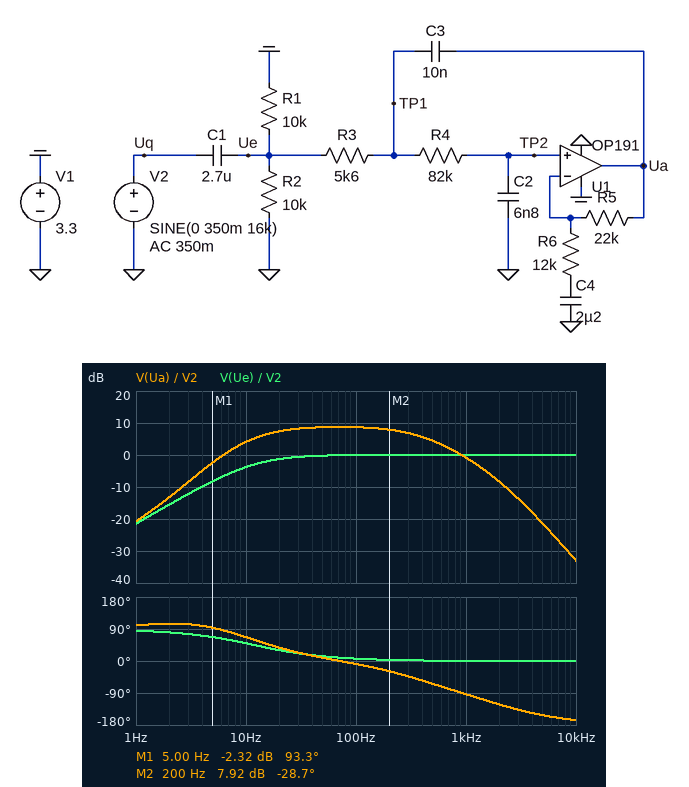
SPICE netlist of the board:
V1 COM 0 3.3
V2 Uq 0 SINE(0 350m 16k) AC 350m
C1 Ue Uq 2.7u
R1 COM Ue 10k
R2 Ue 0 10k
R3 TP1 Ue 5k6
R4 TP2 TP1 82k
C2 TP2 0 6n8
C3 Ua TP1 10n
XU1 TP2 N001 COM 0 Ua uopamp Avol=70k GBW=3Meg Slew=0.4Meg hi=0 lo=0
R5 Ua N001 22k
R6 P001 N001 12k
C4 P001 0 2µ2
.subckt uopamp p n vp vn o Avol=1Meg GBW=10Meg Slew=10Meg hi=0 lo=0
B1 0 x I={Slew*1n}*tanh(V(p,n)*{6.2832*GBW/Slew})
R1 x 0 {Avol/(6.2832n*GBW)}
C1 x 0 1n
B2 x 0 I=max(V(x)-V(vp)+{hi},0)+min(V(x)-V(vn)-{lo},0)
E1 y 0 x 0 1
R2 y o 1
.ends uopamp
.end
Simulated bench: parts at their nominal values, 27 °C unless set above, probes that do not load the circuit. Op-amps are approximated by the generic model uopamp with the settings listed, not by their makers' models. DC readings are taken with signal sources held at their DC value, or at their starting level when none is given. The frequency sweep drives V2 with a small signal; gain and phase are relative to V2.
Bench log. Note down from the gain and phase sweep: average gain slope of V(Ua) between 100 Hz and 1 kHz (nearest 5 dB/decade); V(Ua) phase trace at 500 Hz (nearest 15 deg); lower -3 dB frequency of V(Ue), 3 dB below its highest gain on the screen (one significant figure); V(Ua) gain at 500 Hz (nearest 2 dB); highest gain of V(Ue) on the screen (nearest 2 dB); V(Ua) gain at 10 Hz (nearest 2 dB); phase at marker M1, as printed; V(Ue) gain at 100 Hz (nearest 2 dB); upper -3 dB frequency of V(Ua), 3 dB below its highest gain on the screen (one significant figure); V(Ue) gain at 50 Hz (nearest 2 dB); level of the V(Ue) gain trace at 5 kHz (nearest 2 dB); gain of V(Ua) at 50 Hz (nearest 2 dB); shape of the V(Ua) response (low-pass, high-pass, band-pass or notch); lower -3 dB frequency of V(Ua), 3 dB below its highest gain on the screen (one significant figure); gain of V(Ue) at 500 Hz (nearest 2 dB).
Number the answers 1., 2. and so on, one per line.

1. -10 dB/decade
2. -60 deg
3. 10 Hz
4. 4 dB
5. 0 dB
6. 4 dB
7. 93.3 deg
8. 0 dB
9. 400 Hz
10. 0 dB
11. 0 dB
12. 8 dB
13. band-pass
14. 10 Hz
15. 0 dB
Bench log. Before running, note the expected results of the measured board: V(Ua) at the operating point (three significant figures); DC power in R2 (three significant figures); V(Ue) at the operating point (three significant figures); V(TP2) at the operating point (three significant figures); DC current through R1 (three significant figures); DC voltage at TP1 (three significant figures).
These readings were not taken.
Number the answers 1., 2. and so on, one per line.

1. 1.65 V
2. 272 µW
3. 1.65 V
4. 1.65 V
5. 165 µA
6. 1.65 V
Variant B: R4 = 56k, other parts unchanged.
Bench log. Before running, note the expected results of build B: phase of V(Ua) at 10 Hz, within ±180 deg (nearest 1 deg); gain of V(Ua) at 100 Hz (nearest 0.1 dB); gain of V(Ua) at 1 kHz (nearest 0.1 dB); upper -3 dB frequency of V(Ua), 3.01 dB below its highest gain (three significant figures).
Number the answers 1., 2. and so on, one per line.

1. 68 deg
2. 8.9 dB
3. 3.0 dB
4. 645 Hz
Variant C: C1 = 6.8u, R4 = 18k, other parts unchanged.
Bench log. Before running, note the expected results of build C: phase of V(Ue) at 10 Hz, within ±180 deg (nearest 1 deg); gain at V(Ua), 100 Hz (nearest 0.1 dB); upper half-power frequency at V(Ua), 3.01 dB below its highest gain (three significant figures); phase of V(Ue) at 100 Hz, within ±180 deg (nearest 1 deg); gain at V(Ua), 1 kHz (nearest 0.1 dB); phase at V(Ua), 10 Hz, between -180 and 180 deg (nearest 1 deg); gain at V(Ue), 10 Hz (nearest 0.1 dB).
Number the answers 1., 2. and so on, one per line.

1. 25 deg
2. 9.0 dB
3. 2.28 kHz
4. 3 deg
5. 10.8 dB
6. 44 deg
7. -0.9 dB
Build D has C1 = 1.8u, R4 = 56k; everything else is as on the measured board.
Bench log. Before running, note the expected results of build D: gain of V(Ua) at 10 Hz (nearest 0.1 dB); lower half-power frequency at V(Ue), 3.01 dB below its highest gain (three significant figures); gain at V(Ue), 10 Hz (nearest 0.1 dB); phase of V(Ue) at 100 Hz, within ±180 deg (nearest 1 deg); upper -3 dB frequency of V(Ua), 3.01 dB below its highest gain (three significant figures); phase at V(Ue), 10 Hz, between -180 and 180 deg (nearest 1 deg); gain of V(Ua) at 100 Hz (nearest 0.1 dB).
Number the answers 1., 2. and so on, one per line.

1. 1.7 dB
2. 17.7 Hz
3. -6.2 dB
4. 10 deg
5. 650 Hz
6. 61 deg
7. 8.8 dB
